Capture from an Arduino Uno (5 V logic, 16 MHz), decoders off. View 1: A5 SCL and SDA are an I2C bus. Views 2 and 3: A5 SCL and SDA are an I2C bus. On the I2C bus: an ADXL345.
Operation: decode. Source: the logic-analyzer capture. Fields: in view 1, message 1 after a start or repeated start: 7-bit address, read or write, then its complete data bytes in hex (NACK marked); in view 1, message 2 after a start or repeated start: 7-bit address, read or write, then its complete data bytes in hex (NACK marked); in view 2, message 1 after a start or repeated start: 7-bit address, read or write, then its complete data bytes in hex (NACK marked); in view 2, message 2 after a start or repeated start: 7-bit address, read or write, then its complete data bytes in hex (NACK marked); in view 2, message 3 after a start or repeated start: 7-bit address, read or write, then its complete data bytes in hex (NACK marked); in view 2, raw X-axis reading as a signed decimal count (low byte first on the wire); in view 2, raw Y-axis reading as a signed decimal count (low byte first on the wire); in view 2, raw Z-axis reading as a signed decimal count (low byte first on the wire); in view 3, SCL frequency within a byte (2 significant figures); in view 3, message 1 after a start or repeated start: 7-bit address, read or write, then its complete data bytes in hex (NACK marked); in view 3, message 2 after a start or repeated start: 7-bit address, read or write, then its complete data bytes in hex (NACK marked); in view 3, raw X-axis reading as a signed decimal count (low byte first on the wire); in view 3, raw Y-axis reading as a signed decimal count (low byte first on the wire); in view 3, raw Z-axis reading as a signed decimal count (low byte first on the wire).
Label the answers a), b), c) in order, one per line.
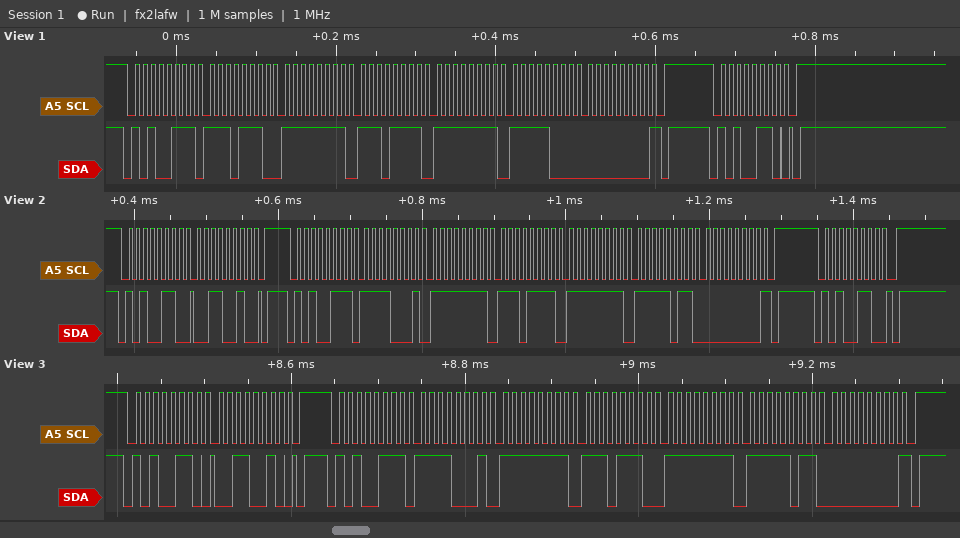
a) 0x53 read: EE FF EF FF F8 00 NACK
b) 0x53 write
c) 0x53 write: 32
d) 0x53 read: F1 FF EF FF FB 00 NACK
e) 0x53 write
f) -15
g) -17
h) 251
i) 100 kHz
j) 0x53 write: 32
k) 0x53 read: F1 FF EE FF FB 00 NACK
l) -15
m) -18
n) 251
